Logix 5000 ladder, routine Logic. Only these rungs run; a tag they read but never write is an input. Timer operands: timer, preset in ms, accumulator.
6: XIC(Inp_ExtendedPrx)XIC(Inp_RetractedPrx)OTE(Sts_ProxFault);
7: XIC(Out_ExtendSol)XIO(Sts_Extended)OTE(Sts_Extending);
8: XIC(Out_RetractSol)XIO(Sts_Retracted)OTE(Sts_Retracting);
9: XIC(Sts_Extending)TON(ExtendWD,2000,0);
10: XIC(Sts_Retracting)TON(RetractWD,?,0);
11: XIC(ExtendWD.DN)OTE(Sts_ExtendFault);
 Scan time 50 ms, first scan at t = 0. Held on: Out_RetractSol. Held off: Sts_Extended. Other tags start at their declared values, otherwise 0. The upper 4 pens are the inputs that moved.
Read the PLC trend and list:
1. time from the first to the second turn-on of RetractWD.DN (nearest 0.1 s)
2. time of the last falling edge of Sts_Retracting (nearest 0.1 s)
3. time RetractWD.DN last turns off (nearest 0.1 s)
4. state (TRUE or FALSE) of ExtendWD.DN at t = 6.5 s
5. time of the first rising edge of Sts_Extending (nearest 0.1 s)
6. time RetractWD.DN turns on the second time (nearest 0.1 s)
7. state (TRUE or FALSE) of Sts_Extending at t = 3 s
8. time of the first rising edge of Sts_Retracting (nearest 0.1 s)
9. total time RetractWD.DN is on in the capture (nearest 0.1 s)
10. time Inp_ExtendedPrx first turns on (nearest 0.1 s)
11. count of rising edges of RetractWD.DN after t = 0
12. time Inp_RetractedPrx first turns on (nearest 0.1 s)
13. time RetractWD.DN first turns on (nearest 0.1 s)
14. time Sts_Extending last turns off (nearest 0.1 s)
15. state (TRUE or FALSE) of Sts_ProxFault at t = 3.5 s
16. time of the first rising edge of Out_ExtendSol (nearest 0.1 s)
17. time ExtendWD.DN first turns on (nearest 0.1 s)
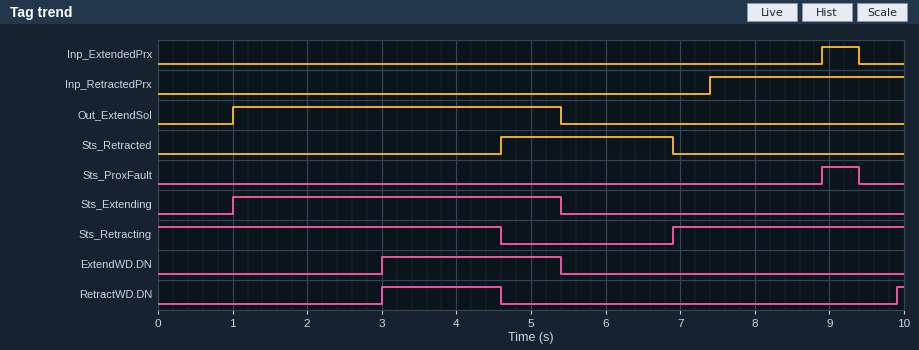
6.9 s
4.6 s
4.6 s
FALSE
1.0 s
9.9 s
TRUE
6.9 s
1.7 s
8.9 s
2
7.4 s
3.0 s
5.4 s
FALSE
1.0 s
3.0 s
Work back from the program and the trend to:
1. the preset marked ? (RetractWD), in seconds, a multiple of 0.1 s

3.0 s
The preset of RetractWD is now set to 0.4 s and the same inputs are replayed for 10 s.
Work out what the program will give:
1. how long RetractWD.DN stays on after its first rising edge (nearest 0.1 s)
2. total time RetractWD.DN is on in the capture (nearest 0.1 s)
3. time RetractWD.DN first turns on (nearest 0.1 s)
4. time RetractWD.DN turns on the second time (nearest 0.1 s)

4.2 s
6.9 s
0.4 s
7.3 s
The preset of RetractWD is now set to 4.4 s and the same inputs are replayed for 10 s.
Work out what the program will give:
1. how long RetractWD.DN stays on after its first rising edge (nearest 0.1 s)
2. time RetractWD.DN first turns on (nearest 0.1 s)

0.2 s
4.4 s
